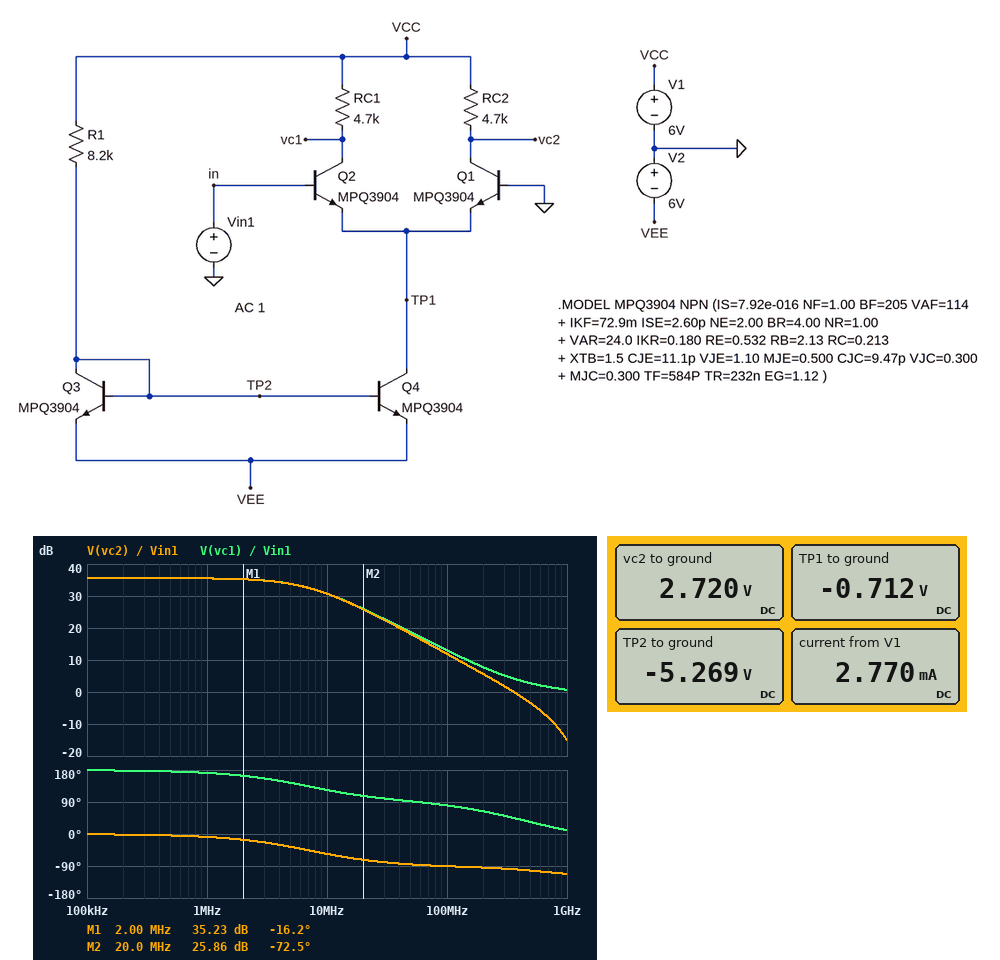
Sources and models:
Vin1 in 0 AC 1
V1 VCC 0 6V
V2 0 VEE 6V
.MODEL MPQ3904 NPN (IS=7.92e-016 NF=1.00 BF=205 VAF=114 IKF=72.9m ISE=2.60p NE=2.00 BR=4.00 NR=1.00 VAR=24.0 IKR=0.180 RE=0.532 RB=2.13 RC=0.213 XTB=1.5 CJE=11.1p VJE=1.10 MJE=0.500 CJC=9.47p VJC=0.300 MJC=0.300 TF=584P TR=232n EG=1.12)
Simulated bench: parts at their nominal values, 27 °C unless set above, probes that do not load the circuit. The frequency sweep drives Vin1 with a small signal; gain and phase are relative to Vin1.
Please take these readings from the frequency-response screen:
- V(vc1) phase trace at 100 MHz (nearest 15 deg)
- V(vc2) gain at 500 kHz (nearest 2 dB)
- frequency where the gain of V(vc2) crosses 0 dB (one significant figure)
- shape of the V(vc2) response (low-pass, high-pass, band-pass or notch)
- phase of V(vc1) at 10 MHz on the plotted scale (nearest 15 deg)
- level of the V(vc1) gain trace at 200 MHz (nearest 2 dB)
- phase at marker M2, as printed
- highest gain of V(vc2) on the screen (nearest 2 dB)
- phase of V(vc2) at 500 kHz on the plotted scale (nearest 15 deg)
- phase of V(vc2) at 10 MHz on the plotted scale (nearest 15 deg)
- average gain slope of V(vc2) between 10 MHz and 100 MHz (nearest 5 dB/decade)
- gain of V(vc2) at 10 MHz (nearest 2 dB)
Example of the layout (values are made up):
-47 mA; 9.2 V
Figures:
75 deg; 36 dB; 400 MHz; low-pass; 120 deg; 8 dB; -72.5 deg; 36 dB; 0 deg; -60 deg; -20 dB/decade; 30 dB
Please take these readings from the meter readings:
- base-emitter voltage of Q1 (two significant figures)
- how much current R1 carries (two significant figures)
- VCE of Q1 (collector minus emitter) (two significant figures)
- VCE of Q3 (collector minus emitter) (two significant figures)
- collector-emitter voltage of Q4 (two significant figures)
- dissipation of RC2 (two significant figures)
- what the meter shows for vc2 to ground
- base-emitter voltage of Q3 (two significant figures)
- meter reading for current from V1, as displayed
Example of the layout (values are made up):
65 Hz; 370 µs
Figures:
710 mV; 1.4 mA; 3.4 V; 730 mV; 5.3 V; 2.3 mW; 2.720 V; 730 mV; 2.770 mA
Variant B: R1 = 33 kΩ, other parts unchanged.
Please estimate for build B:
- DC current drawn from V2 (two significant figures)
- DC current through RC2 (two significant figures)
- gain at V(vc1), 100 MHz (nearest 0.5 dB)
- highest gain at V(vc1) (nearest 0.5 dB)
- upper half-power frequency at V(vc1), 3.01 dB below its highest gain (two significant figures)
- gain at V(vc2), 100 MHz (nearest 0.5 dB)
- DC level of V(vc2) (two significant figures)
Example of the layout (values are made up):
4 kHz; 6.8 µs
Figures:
690 µA; 170 µA; 5.0 dB; 24.0 dB; 8.7 MHz; 1.5 dB; 5.2 V
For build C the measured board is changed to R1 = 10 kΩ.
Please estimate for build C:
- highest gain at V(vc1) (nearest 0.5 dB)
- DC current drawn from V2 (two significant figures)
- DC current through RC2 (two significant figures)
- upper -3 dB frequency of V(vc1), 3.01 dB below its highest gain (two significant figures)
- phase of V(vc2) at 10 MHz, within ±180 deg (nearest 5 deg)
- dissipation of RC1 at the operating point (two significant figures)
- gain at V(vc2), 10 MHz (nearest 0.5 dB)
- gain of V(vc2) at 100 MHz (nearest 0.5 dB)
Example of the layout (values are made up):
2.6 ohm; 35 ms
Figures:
34.0 dB; 2.3 mA; 570 µA; 7.4 MHz; -55 deg; 1.5 mW; 29.5 dB; 10.5 dB
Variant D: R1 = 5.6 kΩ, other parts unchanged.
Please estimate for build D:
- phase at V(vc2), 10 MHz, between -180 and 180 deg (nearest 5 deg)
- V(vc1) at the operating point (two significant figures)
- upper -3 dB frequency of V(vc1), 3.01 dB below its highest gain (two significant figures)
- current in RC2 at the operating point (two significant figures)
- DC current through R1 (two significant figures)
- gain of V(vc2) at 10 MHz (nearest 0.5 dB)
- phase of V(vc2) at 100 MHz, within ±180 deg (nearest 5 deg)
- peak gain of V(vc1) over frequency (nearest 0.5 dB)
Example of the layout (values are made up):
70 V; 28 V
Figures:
-60 deg; 1.2 V; 5.6 MHz; 1.0 mA; 2.0 mA; 32.5 dB; -90 deg; 38.5 dB
